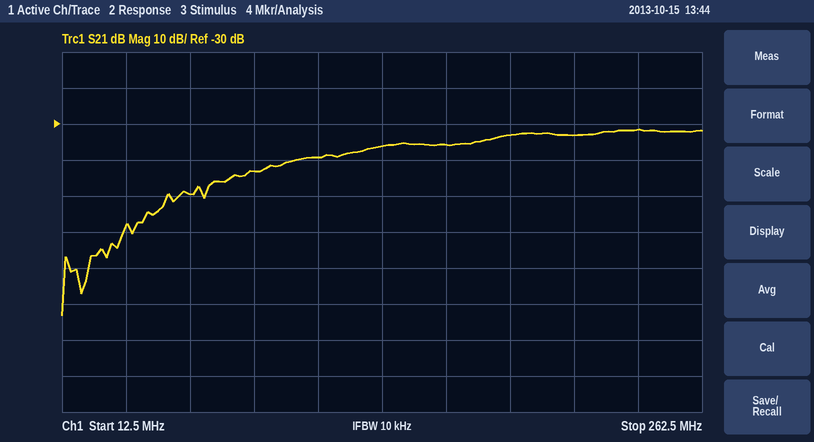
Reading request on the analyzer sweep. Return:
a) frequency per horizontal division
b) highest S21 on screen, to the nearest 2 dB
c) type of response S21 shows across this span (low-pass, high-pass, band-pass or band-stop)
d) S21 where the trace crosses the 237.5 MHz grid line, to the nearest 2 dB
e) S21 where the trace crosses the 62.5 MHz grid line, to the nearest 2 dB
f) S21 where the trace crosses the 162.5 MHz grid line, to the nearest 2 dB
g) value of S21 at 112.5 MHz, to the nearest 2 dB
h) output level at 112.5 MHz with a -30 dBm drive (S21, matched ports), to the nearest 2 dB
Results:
25 MHz
-32 dB
high-pass
-32 dB
-50 dB
-36 dB
-40 dB
-70 dBm
